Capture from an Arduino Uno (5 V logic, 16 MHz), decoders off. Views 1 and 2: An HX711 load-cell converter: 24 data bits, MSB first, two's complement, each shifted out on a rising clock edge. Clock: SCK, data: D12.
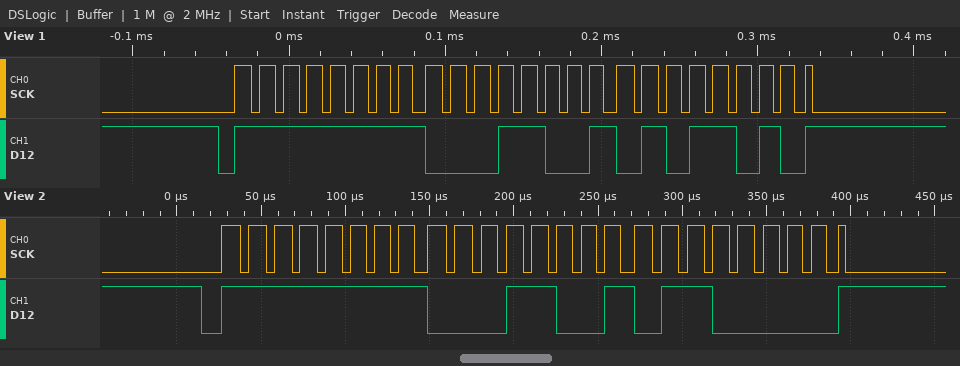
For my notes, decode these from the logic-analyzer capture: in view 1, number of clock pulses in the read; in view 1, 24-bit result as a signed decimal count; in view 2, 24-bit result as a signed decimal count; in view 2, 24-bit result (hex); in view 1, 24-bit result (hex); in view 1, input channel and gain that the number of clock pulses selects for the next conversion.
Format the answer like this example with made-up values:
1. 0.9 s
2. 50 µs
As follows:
1. 25
2. -59046
3. -59040
4. 0xFF1960
5. 0xFF195A
6. channel A, gain 128
